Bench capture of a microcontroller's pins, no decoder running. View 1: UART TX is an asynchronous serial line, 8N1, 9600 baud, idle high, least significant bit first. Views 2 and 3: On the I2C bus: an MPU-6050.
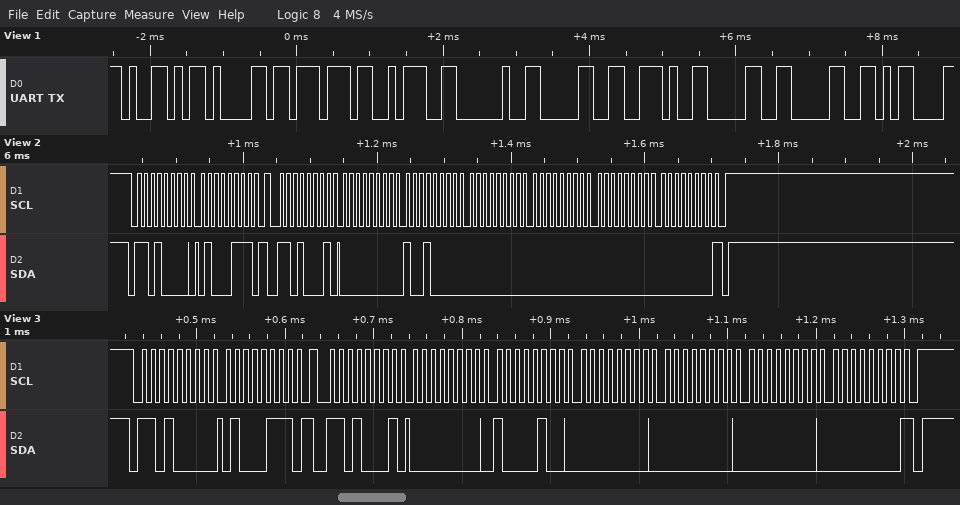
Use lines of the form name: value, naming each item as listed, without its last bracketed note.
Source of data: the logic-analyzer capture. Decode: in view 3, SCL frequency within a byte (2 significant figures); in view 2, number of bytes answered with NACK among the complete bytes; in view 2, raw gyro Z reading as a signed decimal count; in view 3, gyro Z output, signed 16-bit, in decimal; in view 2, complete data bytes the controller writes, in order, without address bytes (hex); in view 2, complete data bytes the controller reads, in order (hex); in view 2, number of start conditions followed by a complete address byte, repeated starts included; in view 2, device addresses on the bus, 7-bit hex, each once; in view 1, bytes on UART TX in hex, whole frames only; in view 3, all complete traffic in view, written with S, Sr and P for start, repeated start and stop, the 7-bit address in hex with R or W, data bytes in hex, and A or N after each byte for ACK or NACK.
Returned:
in view 3, SCL frequency within a byte: 100 kHz
in view 2, number of bytes answered with NACK among the complete bytes: 1
in view 2, raw gyro Z reading as a signed decimal count: 144
in view 3, gyro Z output, signed 16-bit, in decimal: 132
in view 2, complete data bytes the controller writes, in order, without address bytes: 47
in view 2, complete data bytes the controller reads, in order: 00 90 00 00 00 00
in view 2, number of start conditions followed by a complete address byte, repeated starts included: 2
in view 2, device addresses on the bus, 7-bit hex, each once: 0x68
in view 1, bytes on UART TX in hex, whole frames only: 0x59 0x61 0x77 0x3A 0x20 0x30 0x2E 0x30 0x30 0x0D
in view 3, all complete traffic in view, written with S, Sr and P for start, repeated start and stop, the 7-bit address in hex with R or W, data bytes in hex, and A or N after each byte for ACK or NACK: S 68W A 47 A Sr 68R A 00 A 84 A 00 A 00 A 00 A 00 N P
